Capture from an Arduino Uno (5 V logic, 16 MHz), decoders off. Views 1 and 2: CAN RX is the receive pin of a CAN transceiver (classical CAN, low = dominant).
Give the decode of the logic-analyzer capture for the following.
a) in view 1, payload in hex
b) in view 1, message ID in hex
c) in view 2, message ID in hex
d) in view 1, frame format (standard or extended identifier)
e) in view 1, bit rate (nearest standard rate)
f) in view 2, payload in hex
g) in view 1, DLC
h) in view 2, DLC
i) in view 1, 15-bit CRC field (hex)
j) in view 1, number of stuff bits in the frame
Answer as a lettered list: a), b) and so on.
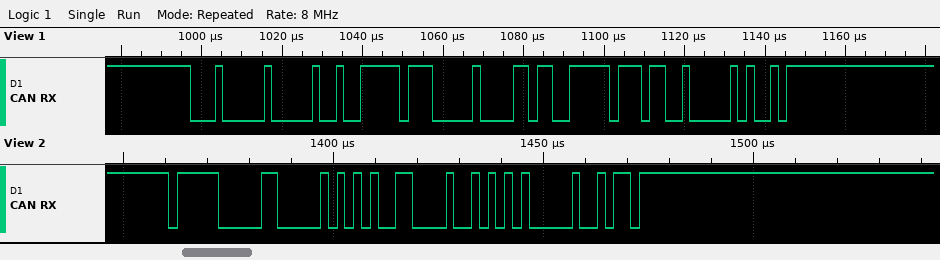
a) FF 00 6C FF
b) 0x100
c) 0x7C2
d) standard
e) 500 kbit/s
f) A6 12
g) 4
h) 2
i) 0x3204
j) 6
